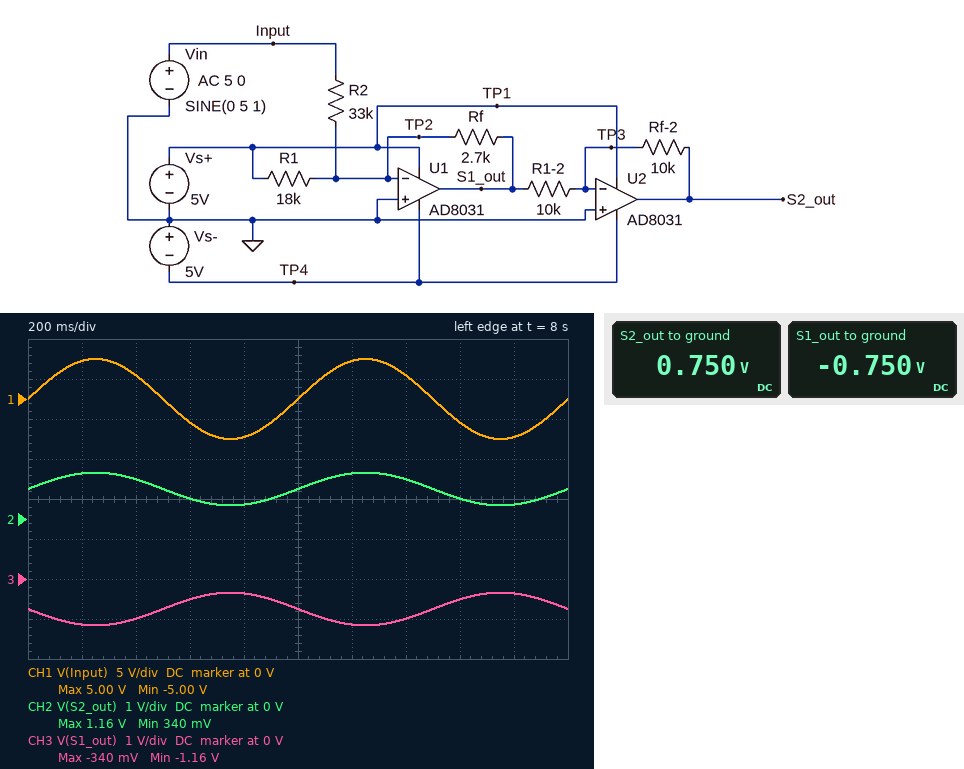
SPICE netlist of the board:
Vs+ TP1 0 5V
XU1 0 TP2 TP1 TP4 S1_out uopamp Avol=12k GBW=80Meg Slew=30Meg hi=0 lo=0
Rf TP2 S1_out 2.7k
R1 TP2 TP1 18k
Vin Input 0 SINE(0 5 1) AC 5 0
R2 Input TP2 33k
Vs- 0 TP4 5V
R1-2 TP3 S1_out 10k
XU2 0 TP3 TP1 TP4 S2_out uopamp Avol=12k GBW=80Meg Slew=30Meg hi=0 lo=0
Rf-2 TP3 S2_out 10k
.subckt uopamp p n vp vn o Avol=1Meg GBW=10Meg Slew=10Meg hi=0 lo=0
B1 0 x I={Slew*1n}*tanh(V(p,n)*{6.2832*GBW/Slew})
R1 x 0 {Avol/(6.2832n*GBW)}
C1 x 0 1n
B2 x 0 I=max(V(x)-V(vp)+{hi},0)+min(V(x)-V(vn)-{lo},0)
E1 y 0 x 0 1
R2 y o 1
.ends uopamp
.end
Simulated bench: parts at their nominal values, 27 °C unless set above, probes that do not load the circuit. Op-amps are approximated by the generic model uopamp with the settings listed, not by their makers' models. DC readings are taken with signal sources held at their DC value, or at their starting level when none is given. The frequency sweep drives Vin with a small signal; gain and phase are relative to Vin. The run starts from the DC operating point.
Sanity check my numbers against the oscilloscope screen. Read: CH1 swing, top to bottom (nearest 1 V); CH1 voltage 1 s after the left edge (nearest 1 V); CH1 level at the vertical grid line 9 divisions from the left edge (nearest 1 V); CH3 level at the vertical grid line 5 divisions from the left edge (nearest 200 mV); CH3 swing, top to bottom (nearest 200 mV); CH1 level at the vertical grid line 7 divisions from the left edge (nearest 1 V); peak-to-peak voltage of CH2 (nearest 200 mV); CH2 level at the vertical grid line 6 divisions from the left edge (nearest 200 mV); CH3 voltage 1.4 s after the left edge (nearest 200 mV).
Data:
10 V
0 V
-5 V
-800 mV
800 mV
3 V
800 mV
1.2 V
-1.0 V
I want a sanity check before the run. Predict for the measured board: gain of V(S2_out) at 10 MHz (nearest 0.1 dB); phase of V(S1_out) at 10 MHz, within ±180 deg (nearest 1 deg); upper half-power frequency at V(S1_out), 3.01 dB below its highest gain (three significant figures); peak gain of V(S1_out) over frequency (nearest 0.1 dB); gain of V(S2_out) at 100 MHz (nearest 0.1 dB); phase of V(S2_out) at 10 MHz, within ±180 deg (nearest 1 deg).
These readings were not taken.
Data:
-22.1 dB
171 deg
64.9 MHz
-21.7 dB
-35.6 dB
-23 deg
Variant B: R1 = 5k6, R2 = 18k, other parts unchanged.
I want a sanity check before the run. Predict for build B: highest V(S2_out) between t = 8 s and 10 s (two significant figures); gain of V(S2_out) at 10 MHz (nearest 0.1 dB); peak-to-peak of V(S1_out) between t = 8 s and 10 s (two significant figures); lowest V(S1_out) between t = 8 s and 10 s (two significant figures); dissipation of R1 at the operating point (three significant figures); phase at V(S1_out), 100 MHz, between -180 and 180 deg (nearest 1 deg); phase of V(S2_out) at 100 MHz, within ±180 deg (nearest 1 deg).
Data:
3.2 V
-16.9 dB
1.5 V
-3.2 V
4.46 mW
116 deg
-132 deg
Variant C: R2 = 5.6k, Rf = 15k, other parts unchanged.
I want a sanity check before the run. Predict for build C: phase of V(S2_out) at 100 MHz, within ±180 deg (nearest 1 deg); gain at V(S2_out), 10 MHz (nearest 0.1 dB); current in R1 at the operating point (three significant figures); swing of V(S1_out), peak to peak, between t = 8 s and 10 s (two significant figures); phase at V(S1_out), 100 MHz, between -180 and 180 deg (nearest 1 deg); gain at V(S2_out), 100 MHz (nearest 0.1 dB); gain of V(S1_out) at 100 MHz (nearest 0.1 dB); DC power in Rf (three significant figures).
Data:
-148 deg
7.1 dB
278 µA
10 V
100 deg
-15.2 dB
-6.6 dB
1.16 mW
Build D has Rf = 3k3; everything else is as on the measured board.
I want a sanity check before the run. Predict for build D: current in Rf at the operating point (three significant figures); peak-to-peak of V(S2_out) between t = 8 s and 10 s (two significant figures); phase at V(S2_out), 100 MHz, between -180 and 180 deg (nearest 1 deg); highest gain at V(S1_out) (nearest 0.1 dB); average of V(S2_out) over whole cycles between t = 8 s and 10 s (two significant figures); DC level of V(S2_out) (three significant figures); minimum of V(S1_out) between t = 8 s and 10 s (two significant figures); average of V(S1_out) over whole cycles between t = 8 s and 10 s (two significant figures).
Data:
278 µA
1.0 V
-126 deg
-20.0 dB
920 mV
916 mV
-1.4 V
-920 mV
